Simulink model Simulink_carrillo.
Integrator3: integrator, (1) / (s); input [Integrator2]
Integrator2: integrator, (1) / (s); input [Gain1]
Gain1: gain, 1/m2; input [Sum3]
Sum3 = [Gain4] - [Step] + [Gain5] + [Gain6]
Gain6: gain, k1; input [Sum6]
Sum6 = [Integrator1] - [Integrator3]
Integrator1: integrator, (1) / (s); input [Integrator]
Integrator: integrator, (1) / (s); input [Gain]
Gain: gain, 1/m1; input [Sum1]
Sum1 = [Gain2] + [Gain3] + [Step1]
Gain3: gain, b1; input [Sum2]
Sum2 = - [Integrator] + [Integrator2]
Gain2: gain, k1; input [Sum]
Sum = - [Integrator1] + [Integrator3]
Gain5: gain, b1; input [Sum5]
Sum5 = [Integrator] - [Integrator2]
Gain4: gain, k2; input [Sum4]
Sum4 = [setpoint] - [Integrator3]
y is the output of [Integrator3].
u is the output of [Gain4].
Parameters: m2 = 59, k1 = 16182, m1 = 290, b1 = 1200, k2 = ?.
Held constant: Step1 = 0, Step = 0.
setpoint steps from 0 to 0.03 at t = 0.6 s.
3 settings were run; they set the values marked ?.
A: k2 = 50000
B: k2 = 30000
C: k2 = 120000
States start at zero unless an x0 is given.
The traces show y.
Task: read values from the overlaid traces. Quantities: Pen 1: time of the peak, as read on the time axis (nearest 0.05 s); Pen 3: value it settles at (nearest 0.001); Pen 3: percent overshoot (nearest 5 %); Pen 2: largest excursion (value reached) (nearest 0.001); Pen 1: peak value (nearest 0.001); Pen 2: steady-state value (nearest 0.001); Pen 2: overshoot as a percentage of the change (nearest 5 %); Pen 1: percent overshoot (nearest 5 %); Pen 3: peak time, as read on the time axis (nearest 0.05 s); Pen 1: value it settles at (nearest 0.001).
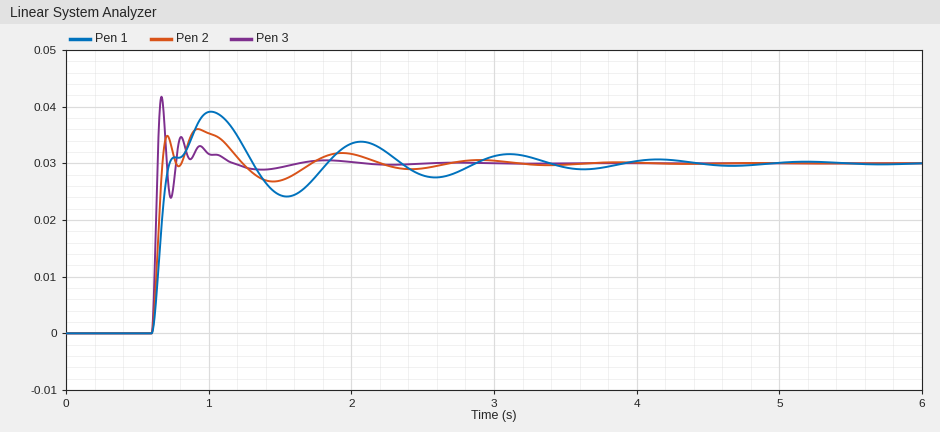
1.00 s
0.030
40 %
0.036
0.039
0.030
20 %
30 %
0.65 s
0.030
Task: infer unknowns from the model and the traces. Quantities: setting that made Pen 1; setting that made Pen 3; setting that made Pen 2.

B
C
A
